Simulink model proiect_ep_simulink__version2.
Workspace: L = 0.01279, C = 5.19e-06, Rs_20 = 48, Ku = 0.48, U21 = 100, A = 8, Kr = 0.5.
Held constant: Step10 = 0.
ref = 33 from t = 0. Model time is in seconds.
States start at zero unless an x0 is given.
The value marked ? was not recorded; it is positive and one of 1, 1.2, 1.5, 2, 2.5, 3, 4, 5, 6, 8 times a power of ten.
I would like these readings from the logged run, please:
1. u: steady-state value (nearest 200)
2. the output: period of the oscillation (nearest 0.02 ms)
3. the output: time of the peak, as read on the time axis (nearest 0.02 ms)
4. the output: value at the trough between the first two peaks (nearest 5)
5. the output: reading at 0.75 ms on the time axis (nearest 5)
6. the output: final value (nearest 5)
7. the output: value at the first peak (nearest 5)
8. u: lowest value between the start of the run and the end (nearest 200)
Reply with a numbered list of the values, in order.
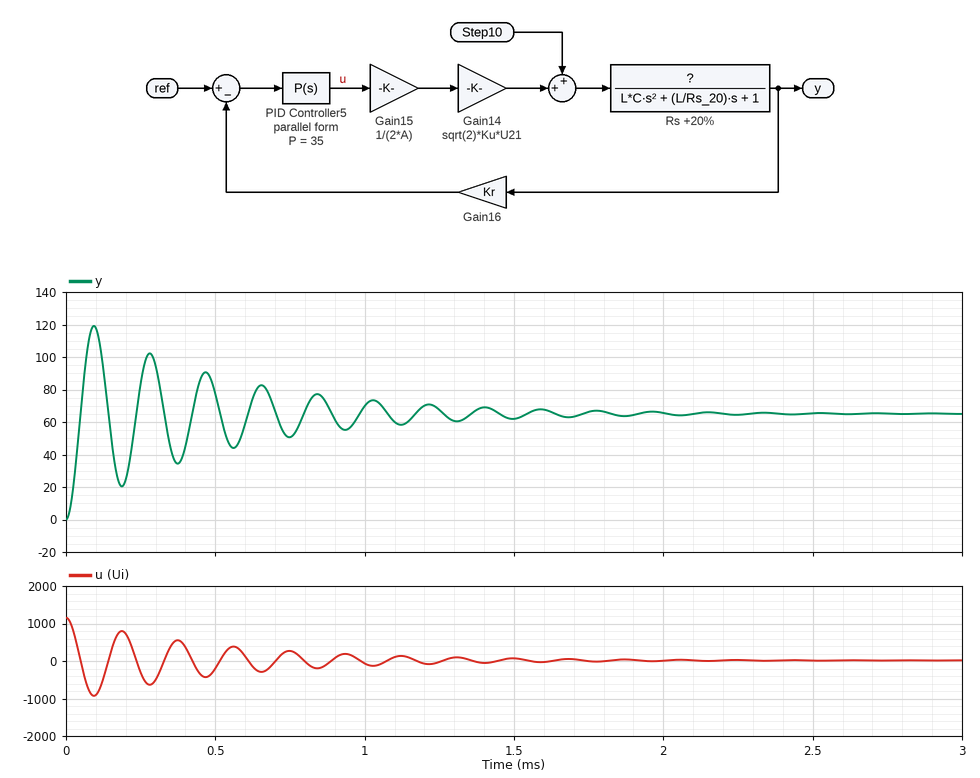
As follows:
1. 0
2. 0.18 ms
3. 0.10 ms
4. 20
5. 50
6. 65
7. 120
8. -1000
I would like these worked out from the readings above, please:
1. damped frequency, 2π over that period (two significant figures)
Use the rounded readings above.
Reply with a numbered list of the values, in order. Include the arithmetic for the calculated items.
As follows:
1. 2π / 0.18 = 35 rad/ms
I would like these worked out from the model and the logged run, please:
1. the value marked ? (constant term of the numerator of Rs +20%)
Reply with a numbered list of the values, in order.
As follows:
1. 1
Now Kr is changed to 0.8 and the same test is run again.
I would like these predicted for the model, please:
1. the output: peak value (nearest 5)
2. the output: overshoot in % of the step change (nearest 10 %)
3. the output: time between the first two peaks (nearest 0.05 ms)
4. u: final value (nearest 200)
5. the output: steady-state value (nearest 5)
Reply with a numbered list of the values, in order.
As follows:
1. 75
2. 90 %
3. 0.15 ms
4. 0
5. 40
